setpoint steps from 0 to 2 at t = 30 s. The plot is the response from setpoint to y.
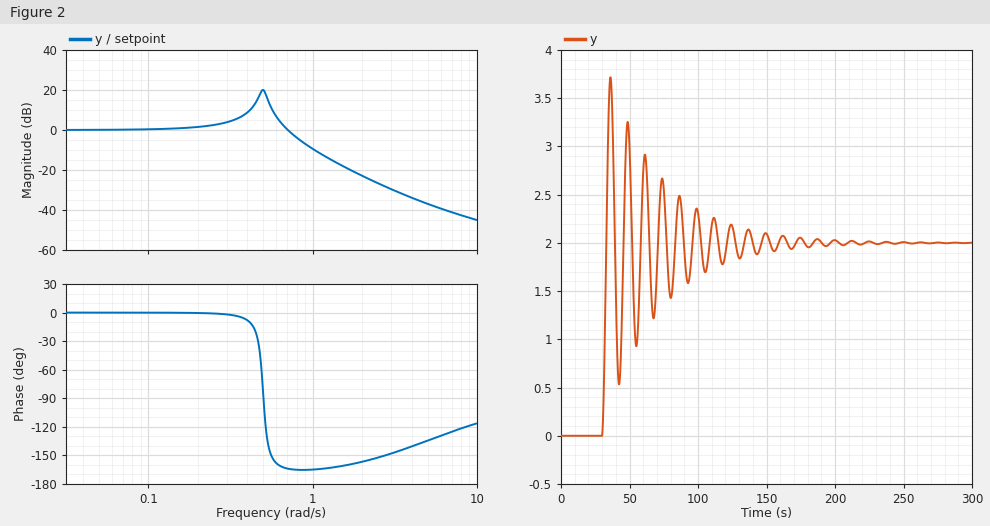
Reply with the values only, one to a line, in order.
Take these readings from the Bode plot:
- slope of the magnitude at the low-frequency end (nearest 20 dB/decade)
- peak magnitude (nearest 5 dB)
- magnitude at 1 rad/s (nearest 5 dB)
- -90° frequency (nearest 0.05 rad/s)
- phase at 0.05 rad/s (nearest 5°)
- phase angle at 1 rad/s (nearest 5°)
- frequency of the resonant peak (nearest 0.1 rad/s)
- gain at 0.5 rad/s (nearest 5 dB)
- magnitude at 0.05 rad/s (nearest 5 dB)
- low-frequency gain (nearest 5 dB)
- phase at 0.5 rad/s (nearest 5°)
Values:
0 dB/decade
20 dB
-10 dB
0.50 rad/s
0°
-165°
0.5 rad/s
20 dB
0 dB
0 dB
-85°
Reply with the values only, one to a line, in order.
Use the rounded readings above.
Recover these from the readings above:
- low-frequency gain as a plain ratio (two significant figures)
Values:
1.0
